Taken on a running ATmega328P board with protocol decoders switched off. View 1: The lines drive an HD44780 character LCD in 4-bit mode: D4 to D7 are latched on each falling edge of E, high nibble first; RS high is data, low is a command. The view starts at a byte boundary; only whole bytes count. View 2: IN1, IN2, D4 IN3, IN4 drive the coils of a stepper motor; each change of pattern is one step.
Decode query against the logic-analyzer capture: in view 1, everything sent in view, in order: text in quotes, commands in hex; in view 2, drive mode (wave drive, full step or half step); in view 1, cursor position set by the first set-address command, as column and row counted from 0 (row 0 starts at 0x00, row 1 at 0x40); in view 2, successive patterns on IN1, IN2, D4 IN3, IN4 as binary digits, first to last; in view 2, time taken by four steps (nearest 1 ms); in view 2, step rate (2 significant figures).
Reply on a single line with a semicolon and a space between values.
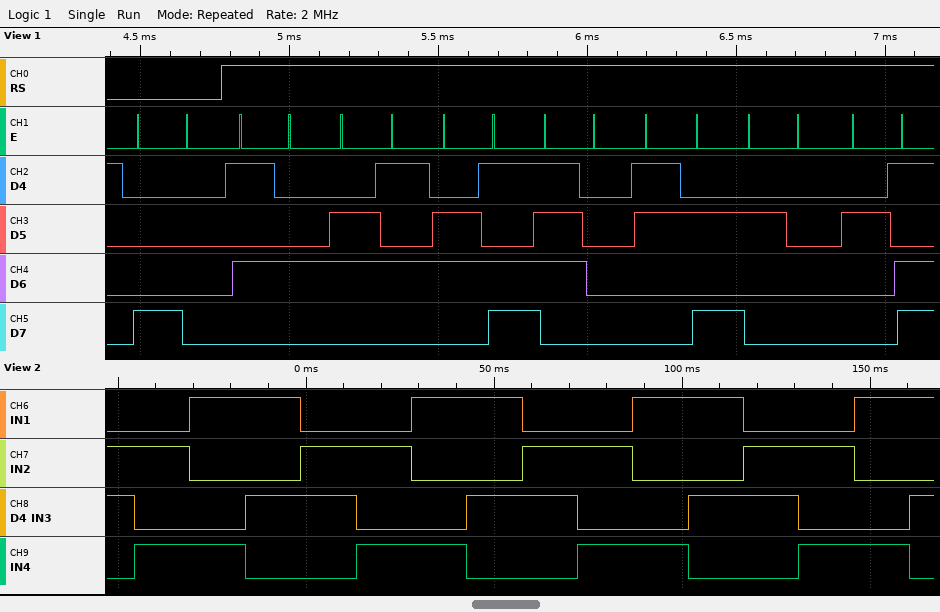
0x80 "Temp: -"; full step; column 0, row 0; 0110 0101 1001 1010 0110 0101 1001 1010 0110 0101 1001 1010 0110 0101 1001 1010; 59 ms; 68 steps/s
